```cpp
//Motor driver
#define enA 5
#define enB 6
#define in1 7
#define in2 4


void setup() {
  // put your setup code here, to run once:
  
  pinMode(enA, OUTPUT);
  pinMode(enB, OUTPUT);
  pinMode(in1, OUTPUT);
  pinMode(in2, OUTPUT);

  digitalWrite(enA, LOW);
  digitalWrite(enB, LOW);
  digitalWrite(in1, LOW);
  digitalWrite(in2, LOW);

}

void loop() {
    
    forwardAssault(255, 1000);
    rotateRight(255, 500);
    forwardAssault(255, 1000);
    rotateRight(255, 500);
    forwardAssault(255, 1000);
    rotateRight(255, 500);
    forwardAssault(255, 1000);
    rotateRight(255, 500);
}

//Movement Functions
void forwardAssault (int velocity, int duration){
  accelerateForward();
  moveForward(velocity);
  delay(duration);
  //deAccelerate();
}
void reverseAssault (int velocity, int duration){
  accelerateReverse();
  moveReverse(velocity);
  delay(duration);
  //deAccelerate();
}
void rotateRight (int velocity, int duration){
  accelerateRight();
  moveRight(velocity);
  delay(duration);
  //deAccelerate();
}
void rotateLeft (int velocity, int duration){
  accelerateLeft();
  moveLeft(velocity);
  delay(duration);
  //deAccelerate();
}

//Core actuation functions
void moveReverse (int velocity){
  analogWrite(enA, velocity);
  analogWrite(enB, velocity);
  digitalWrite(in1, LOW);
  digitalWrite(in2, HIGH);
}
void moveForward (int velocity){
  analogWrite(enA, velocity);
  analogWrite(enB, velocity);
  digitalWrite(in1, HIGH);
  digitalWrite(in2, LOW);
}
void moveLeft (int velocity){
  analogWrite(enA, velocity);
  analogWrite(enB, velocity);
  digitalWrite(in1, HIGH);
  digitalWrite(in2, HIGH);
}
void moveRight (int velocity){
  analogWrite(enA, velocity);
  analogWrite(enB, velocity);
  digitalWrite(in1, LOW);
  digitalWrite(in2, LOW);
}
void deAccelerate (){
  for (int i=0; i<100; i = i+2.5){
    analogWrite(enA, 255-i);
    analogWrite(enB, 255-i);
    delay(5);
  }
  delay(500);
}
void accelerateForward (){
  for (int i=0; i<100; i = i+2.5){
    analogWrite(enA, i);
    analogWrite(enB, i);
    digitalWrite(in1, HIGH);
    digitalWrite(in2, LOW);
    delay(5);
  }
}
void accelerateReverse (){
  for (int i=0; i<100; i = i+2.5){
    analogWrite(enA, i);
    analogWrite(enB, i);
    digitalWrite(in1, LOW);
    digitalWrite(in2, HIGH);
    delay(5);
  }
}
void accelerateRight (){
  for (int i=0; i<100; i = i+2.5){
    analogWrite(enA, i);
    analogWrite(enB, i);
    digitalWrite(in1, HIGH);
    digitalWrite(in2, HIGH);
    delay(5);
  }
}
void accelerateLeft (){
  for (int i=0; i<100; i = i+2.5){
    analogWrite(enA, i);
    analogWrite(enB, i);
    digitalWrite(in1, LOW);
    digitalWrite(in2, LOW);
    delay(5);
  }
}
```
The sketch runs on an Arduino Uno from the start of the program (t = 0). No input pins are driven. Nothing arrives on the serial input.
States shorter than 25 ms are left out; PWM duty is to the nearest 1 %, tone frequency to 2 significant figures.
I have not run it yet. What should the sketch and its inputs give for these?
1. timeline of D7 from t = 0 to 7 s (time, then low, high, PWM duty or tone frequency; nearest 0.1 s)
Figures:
0 s high; 1.5 s low; 2 s high; 3.5 s low; 4 s high; 5.5 s low; 6 s high
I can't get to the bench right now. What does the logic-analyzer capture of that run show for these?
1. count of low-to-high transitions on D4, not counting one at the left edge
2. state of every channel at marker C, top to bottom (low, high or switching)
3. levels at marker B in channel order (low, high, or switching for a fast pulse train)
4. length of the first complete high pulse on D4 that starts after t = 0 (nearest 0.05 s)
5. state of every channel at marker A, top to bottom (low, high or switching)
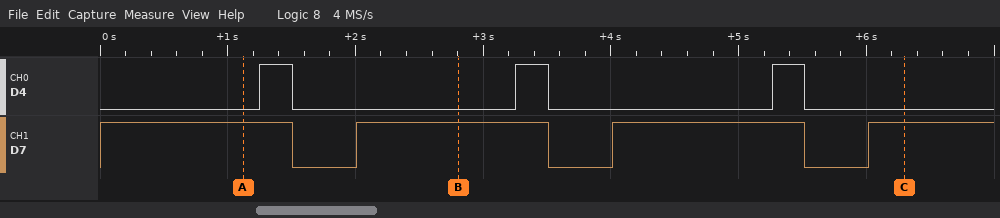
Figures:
3
D4 low, D7 high
D4 low, D7 high
0.25 s
D4 low, D7 high
